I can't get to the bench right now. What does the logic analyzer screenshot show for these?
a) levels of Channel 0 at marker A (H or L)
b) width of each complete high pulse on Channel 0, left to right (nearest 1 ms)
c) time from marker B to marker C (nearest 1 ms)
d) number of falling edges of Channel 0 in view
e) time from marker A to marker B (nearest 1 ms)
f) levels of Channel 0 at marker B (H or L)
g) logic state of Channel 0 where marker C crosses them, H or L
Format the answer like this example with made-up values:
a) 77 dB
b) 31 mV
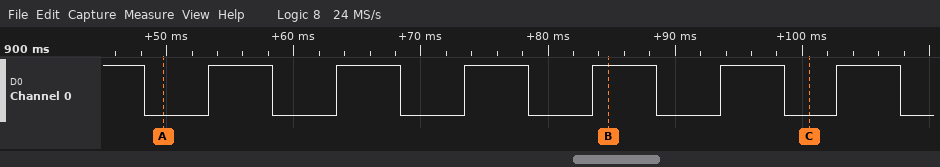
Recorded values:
a) Channel 0=L
b) 5 ms, 5 ms, 5 ms, 5 ms, 5 ms, 5 ms
c) 16 ms
d) 7
e) 35 ms
f) Channel 0=H
g) Channel 0=L
